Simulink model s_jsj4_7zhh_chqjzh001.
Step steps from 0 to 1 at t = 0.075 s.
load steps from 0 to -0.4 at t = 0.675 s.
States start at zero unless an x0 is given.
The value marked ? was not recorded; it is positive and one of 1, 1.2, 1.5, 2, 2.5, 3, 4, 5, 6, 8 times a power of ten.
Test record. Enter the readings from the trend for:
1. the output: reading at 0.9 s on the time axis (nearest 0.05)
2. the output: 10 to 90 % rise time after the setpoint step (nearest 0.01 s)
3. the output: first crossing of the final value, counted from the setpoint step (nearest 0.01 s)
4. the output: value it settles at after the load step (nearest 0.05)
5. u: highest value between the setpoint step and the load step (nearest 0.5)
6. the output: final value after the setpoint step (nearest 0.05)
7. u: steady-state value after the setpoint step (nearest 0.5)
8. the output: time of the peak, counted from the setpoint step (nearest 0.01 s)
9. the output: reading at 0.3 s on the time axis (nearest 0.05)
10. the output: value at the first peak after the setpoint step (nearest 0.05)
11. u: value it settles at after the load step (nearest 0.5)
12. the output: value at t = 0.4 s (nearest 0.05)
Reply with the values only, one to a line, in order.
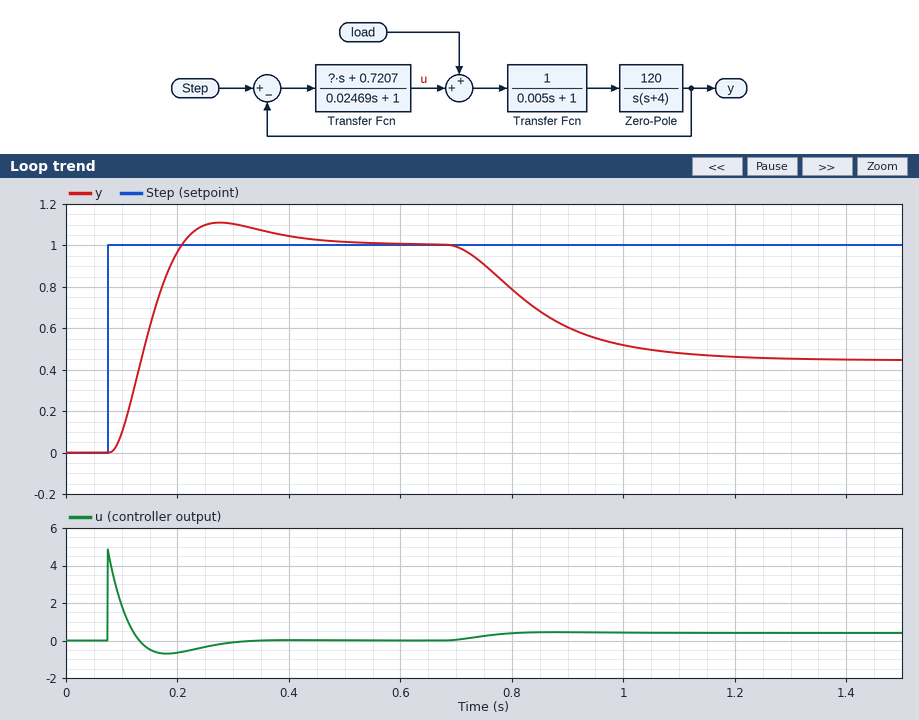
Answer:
0.60
0.09 s
0.13 s
0.45
5.0
1.00
0.0
0.20 s
1.10
1.10
0.5
1.05
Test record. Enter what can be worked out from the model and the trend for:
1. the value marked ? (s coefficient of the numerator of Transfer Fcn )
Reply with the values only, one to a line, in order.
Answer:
0.12
